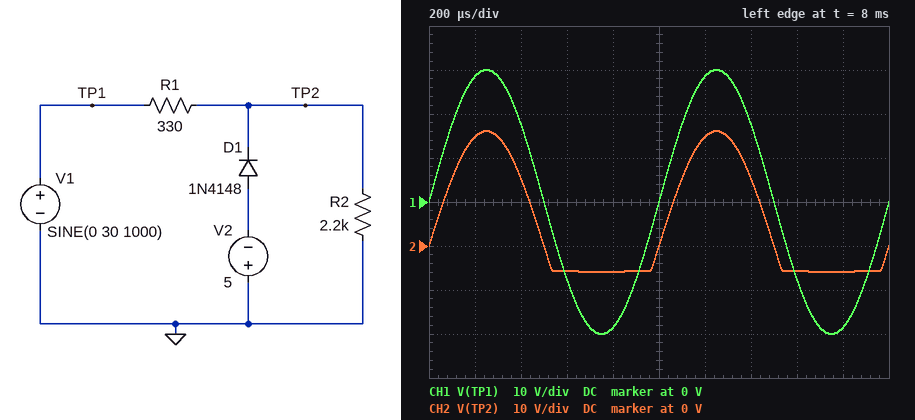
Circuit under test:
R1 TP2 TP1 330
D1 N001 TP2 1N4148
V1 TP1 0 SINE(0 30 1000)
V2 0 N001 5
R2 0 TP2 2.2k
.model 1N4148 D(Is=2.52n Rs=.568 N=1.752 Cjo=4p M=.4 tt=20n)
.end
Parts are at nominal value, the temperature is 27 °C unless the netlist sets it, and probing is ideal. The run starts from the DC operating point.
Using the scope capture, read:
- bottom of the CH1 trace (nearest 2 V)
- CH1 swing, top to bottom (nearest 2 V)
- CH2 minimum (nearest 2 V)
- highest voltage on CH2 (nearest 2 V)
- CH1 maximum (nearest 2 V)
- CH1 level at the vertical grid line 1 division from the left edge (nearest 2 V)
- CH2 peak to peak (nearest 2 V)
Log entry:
-30 V
60 V
-6 V
26 V
30 V
28 V
32 V
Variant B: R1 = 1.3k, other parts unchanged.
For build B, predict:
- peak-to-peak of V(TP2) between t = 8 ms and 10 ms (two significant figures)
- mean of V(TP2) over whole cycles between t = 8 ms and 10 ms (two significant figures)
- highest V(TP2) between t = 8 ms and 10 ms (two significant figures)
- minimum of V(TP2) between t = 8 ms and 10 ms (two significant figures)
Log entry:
25 V
3.4 V
19 V
-5.7 V
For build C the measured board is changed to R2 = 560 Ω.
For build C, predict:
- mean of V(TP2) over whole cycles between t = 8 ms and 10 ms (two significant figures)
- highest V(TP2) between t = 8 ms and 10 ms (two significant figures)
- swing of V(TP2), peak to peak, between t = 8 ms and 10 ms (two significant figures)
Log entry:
3.4 V
19 V
25 V
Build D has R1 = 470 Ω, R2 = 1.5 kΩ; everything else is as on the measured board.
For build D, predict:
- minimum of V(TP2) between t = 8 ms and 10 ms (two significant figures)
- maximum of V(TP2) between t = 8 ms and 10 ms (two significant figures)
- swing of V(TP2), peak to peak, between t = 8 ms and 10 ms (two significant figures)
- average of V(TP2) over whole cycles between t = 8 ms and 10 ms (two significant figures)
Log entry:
-5.8 V
23 V
29 V
4.6 V
